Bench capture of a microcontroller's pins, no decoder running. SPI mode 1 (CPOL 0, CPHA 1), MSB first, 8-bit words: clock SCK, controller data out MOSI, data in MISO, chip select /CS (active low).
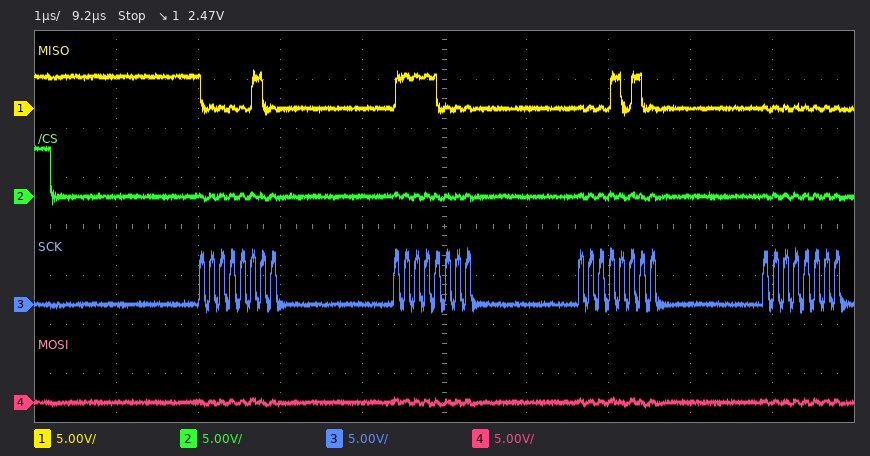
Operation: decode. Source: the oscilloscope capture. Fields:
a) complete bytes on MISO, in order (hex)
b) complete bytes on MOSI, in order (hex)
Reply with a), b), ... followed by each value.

a) 0x04 0xF0 0x14 0x00
b) 0x00 0x00 0x00 0x00
